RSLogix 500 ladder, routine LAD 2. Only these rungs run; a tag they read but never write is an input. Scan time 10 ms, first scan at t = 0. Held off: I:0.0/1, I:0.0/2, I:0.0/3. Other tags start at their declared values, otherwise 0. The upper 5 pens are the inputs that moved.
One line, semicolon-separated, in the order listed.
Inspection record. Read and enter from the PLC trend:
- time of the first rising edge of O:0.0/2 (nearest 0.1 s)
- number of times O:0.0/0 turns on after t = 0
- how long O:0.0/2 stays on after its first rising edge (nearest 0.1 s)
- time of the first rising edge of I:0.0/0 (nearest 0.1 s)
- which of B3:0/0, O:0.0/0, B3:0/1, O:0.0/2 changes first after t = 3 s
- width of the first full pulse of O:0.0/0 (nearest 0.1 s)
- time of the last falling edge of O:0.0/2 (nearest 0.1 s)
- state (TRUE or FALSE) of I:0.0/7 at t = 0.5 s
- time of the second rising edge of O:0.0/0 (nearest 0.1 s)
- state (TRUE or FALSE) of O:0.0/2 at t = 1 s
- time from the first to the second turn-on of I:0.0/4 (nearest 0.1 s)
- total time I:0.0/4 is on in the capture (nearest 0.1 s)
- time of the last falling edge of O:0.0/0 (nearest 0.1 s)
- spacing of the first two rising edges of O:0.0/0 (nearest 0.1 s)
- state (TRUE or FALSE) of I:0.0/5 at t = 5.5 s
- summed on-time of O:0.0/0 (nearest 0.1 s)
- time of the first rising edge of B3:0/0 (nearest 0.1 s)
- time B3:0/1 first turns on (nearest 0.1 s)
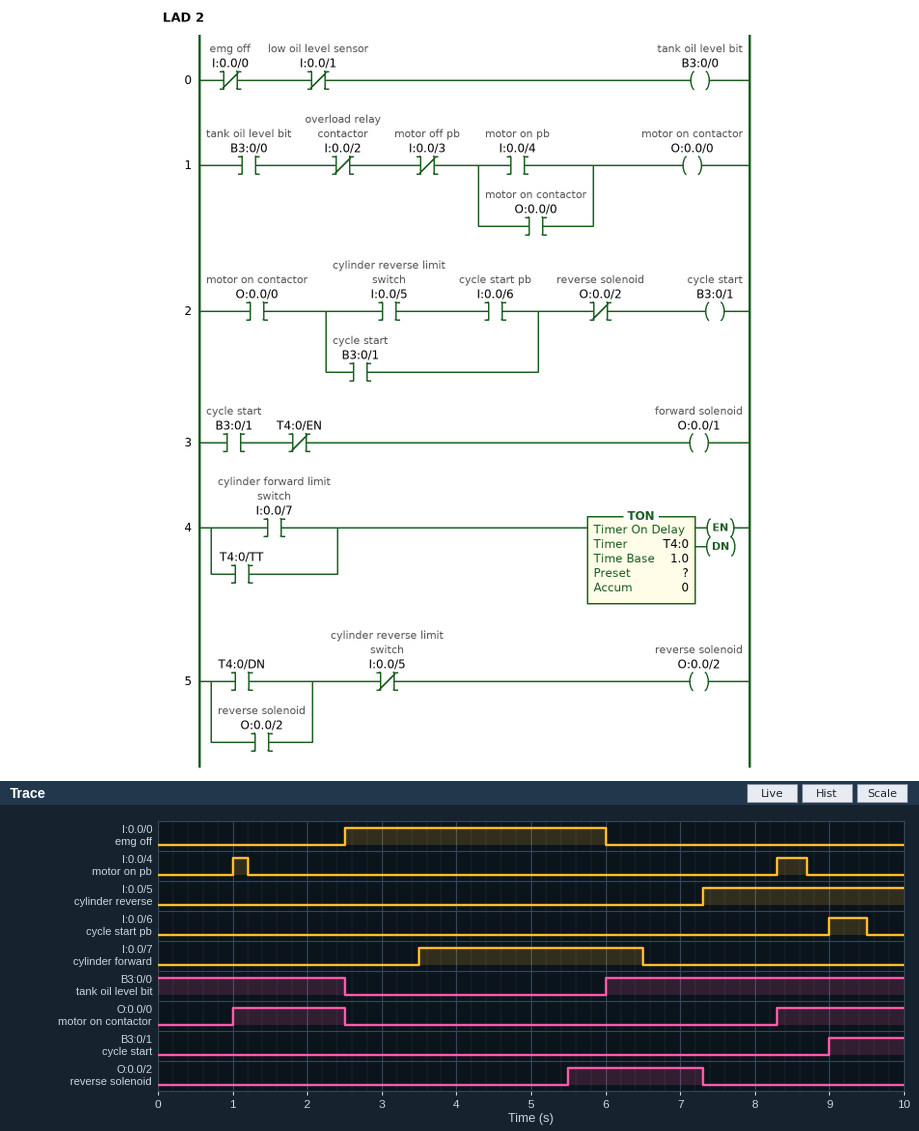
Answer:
5.5 s; 2; 1.8 s; 2.5 s; O:0.0/2; 1.5 s; 7.3 s; FALSE; 8.3 s; FALSE; 7.3 s; 0.6 s; 2.5 s; 7.3 s; FALSE; 3.2 s; 6.0 s; 9.0 s
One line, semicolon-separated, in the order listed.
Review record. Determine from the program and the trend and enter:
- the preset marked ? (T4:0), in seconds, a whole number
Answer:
2 s
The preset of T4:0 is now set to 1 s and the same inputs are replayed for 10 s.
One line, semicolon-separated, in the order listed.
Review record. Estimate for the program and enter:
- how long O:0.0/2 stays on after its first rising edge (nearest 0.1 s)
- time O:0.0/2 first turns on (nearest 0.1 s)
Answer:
2.8 s; 4.5 s
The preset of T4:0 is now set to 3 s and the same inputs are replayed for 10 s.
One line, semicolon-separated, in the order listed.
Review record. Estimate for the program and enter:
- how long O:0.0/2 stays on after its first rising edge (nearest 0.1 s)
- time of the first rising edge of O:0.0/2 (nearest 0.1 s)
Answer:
0.8 s; 6.5 s
